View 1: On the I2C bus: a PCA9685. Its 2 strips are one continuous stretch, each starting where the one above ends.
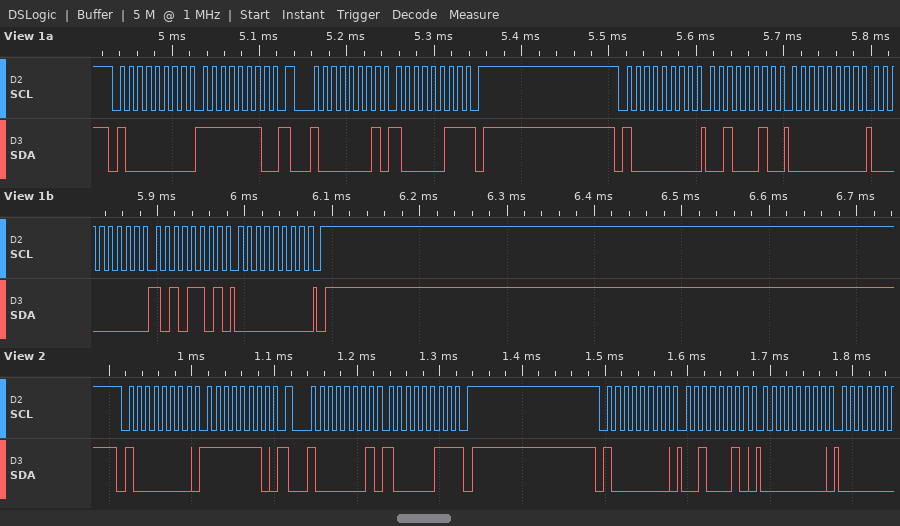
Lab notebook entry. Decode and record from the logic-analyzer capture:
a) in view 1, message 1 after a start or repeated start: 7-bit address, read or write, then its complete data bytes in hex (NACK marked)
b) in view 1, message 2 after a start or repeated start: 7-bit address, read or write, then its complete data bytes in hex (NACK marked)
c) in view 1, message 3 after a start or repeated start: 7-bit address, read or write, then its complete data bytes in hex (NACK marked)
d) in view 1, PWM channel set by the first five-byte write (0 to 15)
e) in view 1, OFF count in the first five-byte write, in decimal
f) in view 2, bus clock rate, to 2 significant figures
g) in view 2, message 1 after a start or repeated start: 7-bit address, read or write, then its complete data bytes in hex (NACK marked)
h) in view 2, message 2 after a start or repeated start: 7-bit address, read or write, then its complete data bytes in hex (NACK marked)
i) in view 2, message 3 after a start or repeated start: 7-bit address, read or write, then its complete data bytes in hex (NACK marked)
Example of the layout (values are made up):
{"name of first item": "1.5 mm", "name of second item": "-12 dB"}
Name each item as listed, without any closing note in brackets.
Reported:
{"in view 1, message 1 after a start or repeated start: 7-bit address, read or write, then its complete data bytes in hex": "0x40 write: FE", "in view 1, message 2 after a start or repeated start: 7-bit address, read or write, then its complete data bytes in hex": "0x40 read: 83 NACK", "in view 1, message 3 after a start or repeated start: 7-bit address, read or write, then its complete data bytes in hex": "0x40 write: 22 00 00 AD 00", "in view 1, PWM channel set by the first five-byte write": "7", "in view 1, OFF count in the first five-byte write, in decimal": "173", "in view 2, bus clock rate, to 2 significant figures": "100 kHz", "in view 2, message 1 after a start or repeated start: 7-bit address, read or write, then its complete data bytes in hex": "0x40 write: FE", "in view 2, message 2 after a start or repeated start: 7-bit address, read or write, then its complete data bytes in hex": "0x40 read: 83 NACK", "in view 2, message 3 after a start or repeated start: 7-bit address, read or write, then its complete data bytes in hex": "0x40 write: 22 00"}
